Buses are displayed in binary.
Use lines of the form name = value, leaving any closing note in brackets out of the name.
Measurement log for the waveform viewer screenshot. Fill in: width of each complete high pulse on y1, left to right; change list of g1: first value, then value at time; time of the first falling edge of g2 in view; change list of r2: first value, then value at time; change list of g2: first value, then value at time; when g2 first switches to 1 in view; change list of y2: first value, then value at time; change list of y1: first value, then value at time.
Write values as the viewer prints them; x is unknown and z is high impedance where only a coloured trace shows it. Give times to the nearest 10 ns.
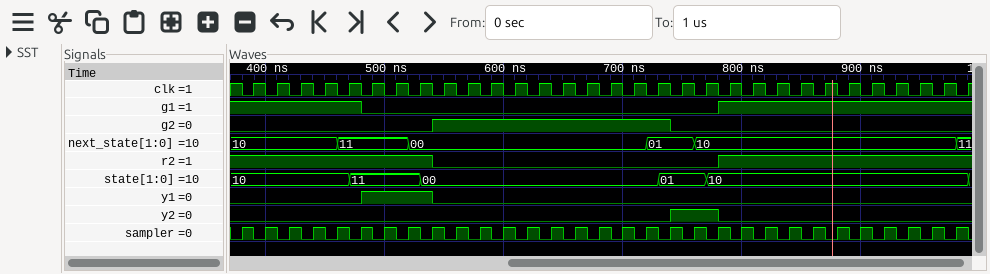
width of each complete high pulse on y1, left to right = 60 ns
change list of g1: first value, then value at time = 1, 0 at 480 ns, 1 at 780 ns
time of the first falling edge of g2 in view = 740 ns
change list of r2: first value, then value at time = 1, 0 at 540 ns, 1 at 780 ns
change list of g2: first value, then value at time = 0, 1 at 540 ns, 0 at 740 ns
when g2 first switches to 1 in view = 540 ns
change list of y2: first value, then value at time = 0, 1 at 740 ns, 0 at 780 ns
change list of y1: first value, then value at time = 0, 1 at 480 ns, 0 at 540 ns
